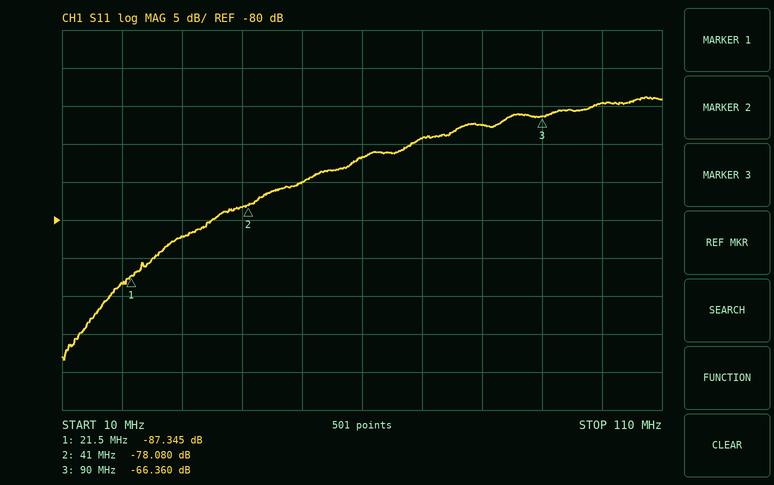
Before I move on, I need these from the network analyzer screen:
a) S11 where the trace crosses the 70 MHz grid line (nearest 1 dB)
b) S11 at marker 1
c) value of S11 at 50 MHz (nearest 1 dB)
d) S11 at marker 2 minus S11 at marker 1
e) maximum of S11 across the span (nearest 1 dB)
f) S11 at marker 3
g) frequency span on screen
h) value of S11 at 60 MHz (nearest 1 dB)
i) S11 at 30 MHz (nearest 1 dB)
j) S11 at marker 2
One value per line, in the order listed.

-69 dB
-87.345 dB
-75 dB
9.265 dB
-64 dB
-66.360 dB
100 MHz
-72 dB
-82 dB
-78.080 dB
